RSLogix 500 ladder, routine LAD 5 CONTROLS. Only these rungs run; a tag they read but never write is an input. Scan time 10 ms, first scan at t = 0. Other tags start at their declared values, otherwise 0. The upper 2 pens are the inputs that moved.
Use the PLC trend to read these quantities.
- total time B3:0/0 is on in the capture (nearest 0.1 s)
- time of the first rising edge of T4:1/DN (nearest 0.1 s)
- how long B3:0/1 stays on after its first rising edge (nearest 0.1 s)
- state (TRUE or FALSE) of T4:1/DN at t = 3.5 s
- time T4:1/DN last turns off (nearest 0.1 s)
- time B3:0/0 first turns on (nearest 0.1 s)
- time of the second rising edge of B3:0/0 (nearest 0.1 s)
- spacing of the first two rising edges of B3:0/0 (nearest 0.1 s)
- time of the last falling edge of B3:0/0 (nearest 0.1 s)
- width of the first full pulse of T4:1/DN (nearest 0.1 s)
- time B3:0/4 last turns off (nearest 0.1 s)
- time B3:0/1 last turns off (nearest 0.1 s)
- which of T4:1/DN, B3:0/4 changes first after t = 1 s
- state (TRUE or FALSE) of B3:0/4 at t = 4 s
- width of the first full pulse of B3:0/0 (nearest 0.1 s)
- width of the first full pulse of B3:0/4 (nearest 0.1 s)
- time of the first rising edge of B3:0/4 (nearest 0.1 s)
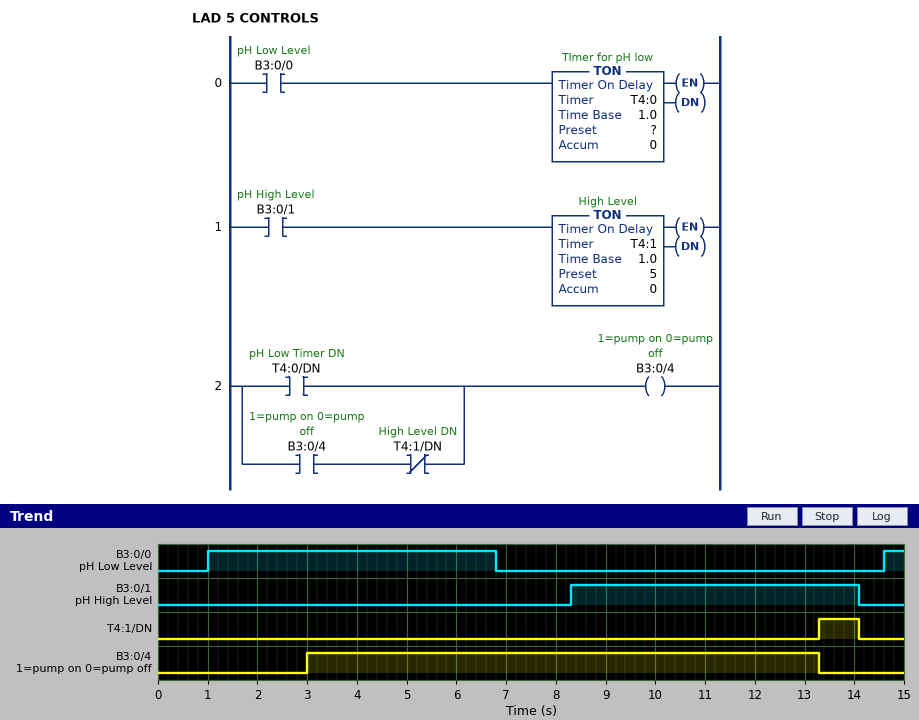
6.2 s
13.3 s
5.8 s
FALSE
14.1 s
1.0 s
14.6 s
13.6 s
6.8 s
0.8 s
13.3 s
14.1 s
B3:0/4
TRUE
5.8 s
10.3 s
3.0 s
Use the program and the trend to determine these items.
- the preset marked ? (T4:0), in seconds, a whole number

2 s
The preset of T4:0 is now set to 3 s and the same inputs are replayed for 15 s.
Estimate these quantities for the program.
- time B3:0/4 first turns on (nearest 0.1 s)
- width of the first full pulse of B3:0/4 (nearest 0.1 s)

4.0 s
9.3 s
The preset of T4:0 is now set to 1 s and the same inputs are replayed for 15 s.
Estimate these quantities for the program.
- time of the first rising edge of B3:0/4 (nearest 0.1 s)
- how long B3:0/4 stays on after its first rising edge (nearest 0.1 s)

2.0 s
11.3 s
